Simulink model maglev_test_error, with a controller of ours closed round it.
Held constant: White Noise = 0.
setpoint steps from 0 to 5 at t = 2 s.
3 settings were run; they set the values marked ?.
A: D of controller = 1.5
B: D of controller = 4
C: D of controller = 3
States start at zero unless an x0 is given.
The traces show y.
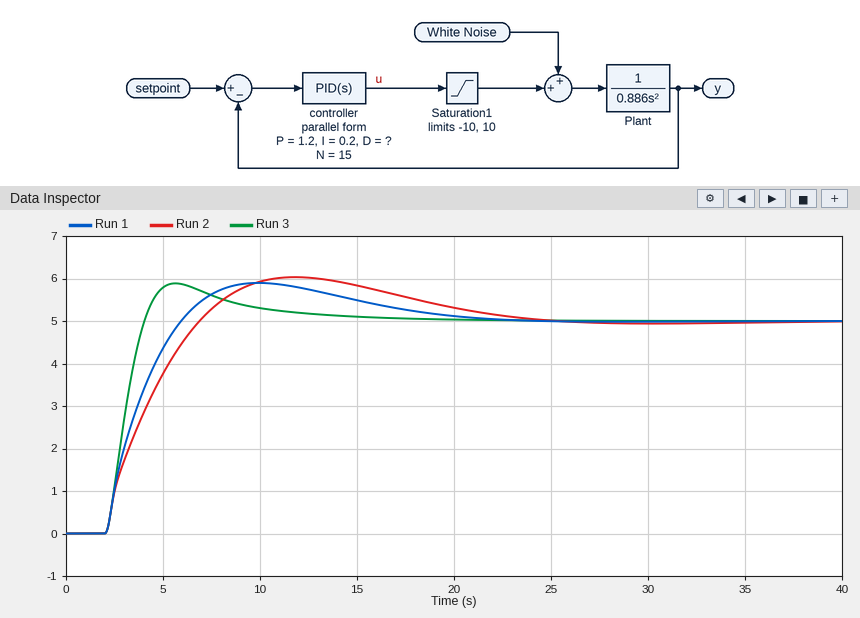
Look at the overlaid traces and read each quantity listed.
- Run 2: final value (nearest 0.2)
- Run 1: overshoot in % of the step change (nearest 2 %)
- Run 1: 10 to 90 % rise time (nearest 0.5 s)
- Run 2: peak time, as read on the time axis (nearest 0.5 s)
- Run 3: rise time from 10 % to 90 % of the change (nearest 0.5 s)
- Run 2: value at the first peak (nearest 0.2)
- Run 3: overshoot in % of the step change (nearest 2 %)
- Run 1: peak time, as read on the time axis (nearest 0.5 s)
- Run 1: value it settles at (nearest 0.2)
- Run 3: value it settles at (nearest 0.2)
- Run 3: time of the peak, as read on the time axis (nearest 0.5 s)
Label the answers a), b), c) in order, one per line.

a) 5.0
b) 18 %
c) 3.0 s
d) 12.0 s
e) 1.5 s
f) 6.0
g) 18 %
h) 10.0 s
i) 5.0
j) 5.0
k) 5.5 s
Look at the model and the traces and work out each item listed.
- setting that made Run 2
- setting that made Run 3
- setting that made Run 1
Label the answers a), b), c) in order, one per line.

a) B
b) A
c) C
